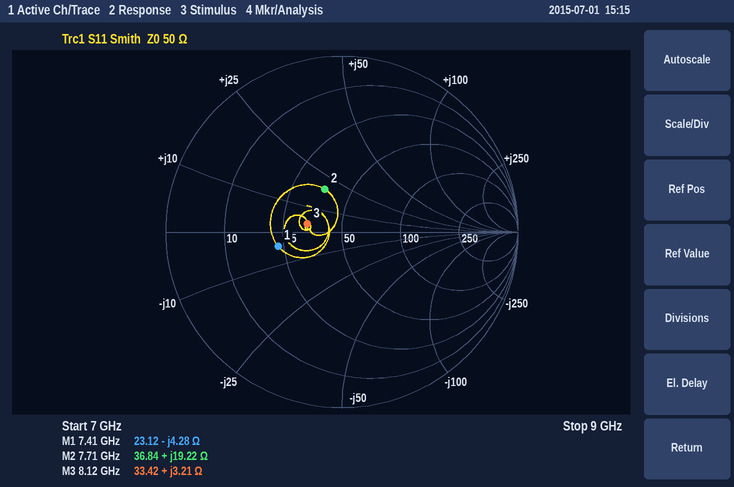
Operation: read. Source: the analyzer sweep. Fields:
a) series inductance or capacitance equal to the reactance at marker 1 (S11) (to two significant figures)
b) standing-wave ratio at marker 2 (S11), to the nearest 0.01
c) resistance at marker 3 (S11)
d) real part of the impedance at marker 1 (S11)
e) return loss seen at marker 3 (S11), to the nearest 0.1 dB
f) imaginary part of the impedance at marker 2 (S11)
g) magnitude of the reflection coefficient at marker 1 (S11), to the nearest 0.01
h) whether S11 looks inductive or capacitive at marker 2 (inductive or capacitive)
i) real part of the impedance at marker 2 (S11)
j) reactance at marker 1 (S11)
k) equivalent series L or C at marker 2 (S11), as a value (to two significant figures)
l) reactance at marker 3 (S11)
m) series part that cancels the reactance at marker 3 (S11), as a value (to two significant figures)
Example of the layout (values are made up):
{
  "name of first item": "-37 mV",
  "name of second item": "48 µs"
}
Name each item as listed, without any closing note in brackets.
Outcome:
{
  "series inductance or capacitance equal to the reactance at marker 1 (S11)": "5.0 pF",
  "standing-wave ratio at marker 2 (S11), to the nearest 0.01": "1.71",
  "resistance at marker 3": "33.42 Ω",
  "real part of the impedance at marker 1": "23.12 Ω",
  "return loss seen at marker 3 (S11), to the nearest 0.1 dB": "13.9 dB",
  "imaginary part of the impedance at marker 2": "+19.22 Ω",
  "magnitude of the reflection coefficient at marker 1 (S11), to the nearest 0.01": "0.37",
  "whether S11 looks inductive or capacitive at marker 2": "inductive",
  "real part of the impedance at marker 2": "36.84 Ω",
  "reactance at marker 1": "-4.28 Ω",
  "equivalent series L or C at marker 2 (S11), as a value": "400 pH",
  "reactance at marker 3": "+3.21 Ω",
  "series part that cancels the reactance at marker 3 (S11), as a value": "6.1 pF"
}
